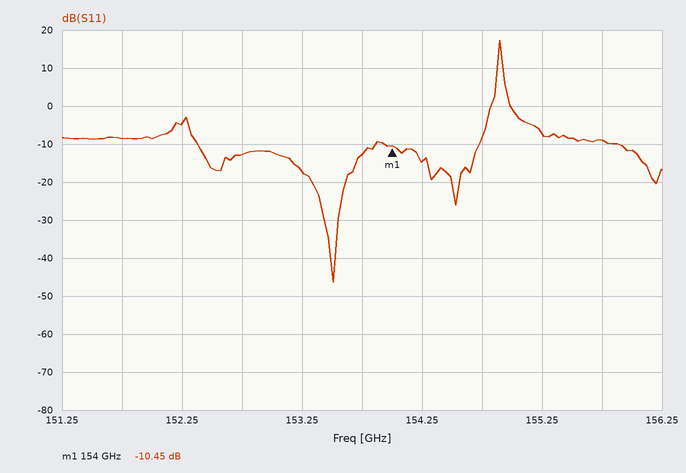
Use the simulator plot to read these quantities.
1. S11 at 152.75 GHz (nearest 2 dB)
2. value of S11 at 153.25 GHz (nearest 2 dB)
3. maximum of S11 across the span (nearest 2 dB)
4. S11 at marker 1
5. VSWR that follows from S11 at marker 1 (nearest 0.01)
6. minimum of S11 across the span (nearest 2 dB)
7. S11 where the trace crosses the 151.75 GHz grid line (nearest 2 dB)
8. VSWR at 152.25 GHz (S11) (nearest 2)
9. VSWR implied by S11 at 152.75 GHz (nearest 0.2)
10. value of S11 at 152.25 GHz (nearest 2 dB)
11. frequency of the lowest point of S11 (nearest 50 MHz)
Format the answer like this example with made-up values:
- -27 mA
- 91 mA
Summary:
- -12 dB
- -18 dB
- 18 dB
- -10.45 dB
- 1.86
- -46 dB
- -8 dB
- 4
- 1.6
- -4 dB
- 153.50 GHz
